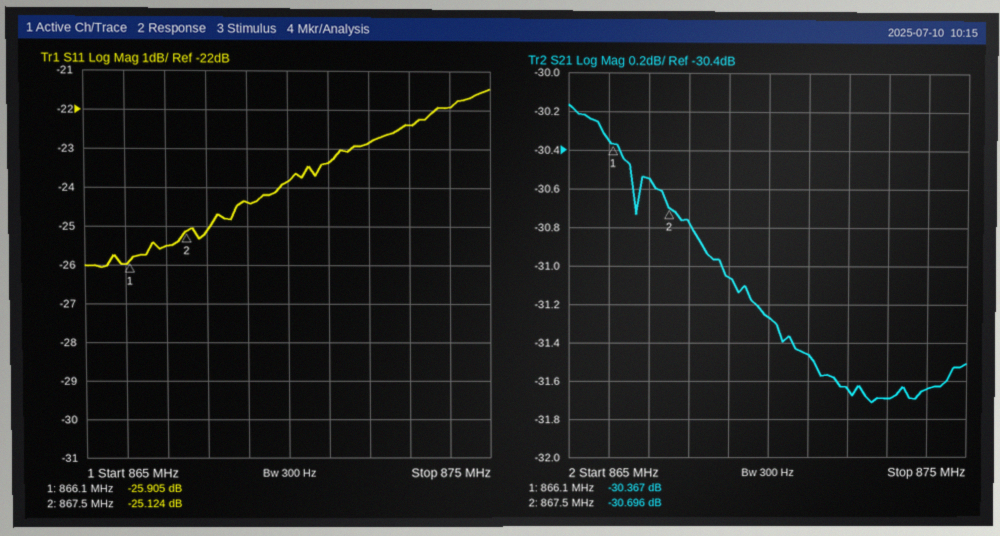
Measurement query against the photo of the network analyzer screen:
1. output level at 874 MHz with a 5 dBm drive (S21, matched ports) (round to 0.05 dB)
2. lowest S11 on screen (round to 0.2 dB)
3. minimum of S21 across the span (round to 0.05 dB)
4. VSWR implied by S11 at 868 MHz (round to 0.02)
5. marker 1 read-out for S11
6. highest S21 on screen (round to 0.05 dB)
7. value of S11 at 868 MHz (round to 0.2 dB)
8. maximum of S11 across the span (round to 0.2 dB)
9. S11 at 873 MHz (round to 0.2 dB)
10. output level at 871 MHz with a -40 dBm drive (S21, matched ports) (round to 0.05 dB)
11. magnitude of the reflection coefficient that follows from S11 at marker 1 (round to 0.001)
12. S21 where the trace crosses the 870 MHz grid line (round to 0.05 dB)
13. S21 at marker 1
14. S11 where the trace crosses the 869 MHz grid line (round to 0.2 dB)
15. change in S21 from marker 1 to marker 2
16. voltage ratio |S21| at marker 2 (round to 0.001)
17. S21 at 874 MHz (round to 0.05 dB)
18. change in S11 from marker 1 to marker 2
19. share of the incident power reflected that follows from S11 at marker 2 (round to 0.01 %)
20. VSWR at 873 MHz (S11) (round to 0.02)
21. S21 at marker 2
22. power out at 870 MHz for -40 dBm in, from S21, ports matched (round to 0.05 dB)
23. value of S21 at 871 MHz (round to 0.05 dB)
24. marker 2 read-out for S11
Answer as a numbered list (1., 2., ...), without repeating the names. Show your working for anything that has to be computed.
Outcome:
1. 5 dBm + (-31.65 dB) = -26.65 dBm
2. -26.0 dB
3. -31.70 dB
4. |Γ| = 10^(-25.2/20) = 0.0550; VSWR = (1 + 0.0550)/(1 − 0.0550) ≈ 1.12
5. -25.905 dB
6. -30.15 dB
7. -25.2 dB
8. -21.4 dB
9. -22.4 dB
10. -40 dBm + (-31.45 dB) = -71.45 dBm
11. 10^(-25.905/20) ≈ 0.051
12. -31.25 dB
13. -30.367 dB
14. -24.4 dB
15. -30.696 − (-30.367) = -0.329 dB
16. 10^(-30.696/20) ≈ 0.029
17. -31.65 dB
18. -25.124 − (-25.905) = 0.781 dB
19. 10^(-25.124/10) ≈ 0.31 %
20. |Γ| = 10^(-22.4/20) = 0.0759; VSWR = (1 + 0.0759)/(1 − 0.0759) ≈ 1.16
21. -30.696 dB
22. -40 dBm + (-31.25 dB) = -71.25 dBm
23. -31.45 dB
24. -25.124 dB
